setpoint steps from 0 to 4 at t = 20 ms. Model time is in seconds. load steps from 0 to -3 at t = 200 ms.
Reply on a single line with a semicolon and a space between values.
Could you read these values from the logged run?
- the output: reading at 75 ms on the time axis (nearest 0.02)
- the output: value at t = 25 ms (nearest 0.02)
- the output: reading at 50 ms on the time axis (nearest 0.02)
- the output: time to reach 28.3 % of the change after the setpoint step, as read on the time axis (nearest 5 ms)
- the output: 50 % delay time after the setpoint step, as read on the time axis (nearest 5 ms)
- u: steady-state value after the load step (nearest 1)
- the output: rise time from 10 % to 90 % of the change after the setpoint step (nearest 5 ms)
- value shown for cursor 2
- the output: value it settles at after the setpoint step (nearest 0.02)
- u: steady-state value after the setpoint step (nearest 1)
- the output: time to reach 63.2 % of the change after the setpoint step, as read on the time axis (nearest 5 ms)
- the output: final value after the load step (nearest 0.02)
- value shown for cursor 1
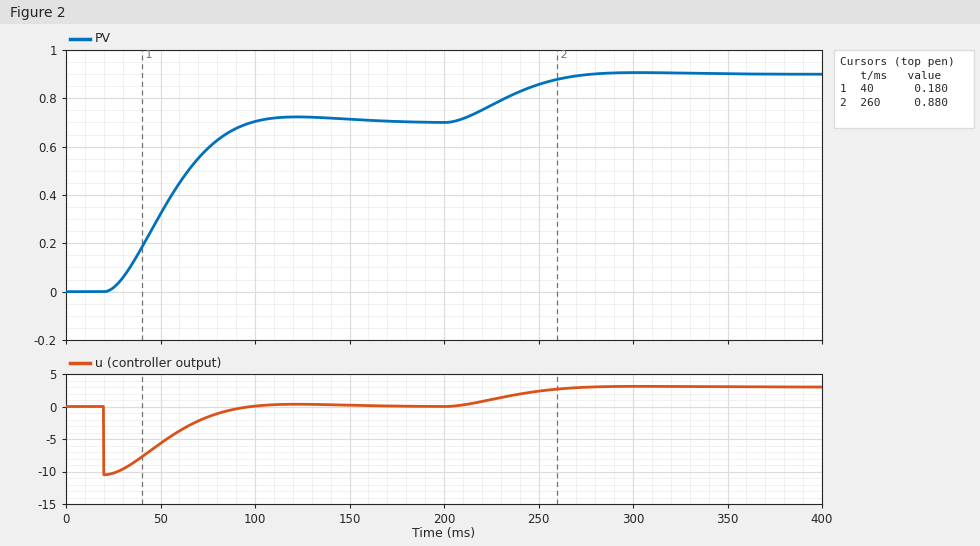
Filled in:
0.60; 0.02; 0.32; 40 ms; 50 ms; 3; 50 ms; 0.880; 0.70; 0; 60 ms; 0.90; 0.180
